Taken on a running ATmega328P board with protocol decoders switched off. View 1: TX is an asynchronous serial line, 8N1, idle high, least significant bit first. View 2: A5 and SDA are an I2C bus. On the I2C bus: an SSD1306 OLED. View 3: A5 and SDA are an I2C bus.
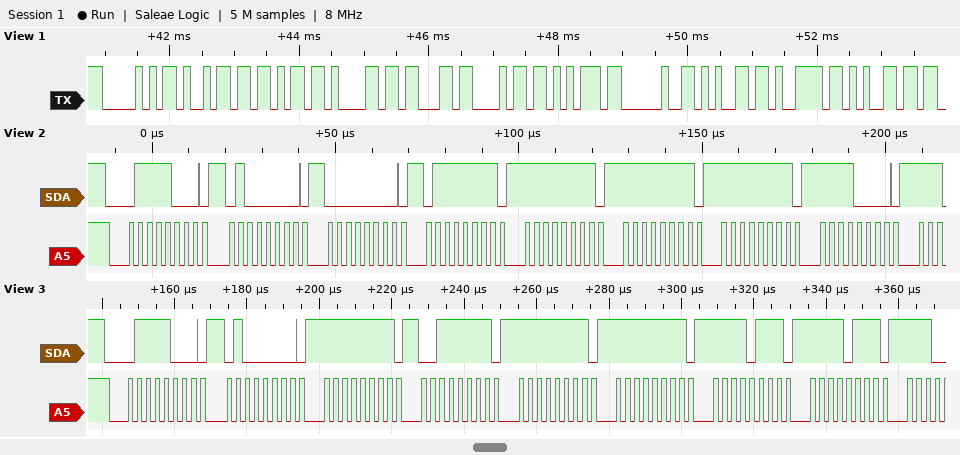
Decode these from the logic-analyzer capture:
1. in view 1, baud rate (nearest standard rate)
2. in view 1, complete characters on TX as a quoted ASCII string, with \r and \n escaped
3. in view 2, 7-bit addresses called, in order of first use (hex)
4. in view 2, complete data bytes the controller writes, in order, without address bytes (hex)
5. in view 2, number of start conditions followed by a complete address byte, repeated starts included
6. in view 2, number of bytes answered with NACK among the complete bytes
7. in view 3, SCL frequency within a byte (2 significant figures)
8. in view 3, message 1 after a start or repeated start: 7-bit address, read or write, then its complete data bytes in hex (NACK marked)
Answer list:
9600 baud
"Pikachu eye"
0x3C
40 00 7F FF FF FF F0
1
0
400 kHz
0x3C write: 40 FF 3F FF FF F7 F7
